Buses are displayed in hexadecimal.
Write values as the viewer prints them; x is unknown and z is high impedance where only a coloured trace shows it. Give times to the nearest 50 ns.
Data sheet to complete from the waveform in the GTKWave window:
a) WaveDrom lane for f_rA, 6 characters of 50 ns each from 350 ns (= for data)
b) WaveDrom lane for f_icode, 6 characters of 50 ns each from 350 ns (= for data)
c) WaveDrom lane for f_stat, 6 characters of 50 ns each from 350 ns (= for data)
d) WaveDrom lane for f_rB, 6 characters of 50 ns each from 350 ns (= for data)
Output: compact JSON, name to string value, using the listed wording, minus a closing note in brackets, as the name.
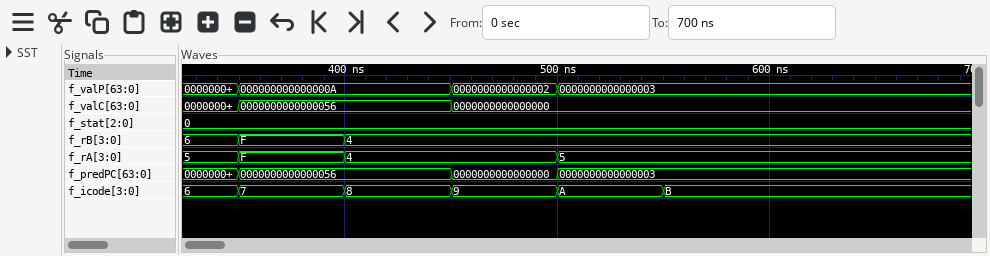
{"WaveDrom lane for f_rA, 6 characters of 50 ns each from 350 ns": "{name: 'f_rA', wave: '==.=..', data: 'F 4 5'}", "WaveDrom lane for f_icode, 6 characters of 50 ns each from 350 ns": "{name: 'f_icode', wave: '=====.', data: '7 8 9 A B'}", "WaveDrom lane for f_stat, 6 characters of 50 ns each from 350 ns": "{name: 'f_stat', wave: '=.....', data: '0'}", "WaveDrom lane for f_rB, 6 characters of 50 ns each from 350 ns": "{name: 'f_rB', wave: '==....', data: 'F 4'}"}
